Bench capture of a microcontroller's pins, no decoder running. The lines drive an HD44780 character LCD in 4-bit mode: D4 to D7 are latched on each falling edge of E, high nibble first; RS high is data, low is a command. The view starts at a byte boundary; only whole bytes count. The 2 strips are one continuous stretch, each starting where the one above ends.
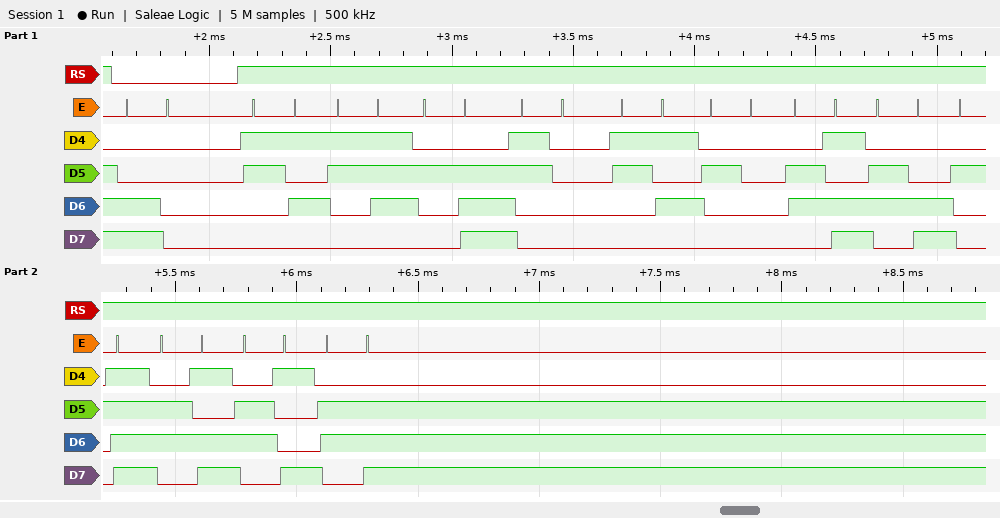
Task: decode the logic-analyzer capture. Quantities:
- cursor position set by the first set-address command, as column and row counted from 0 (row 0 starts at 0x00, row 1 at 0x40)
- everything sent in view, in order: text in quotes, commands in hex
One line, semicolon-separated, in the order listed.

column 0, row 1; 0xC0 "57.05 ml/min"
